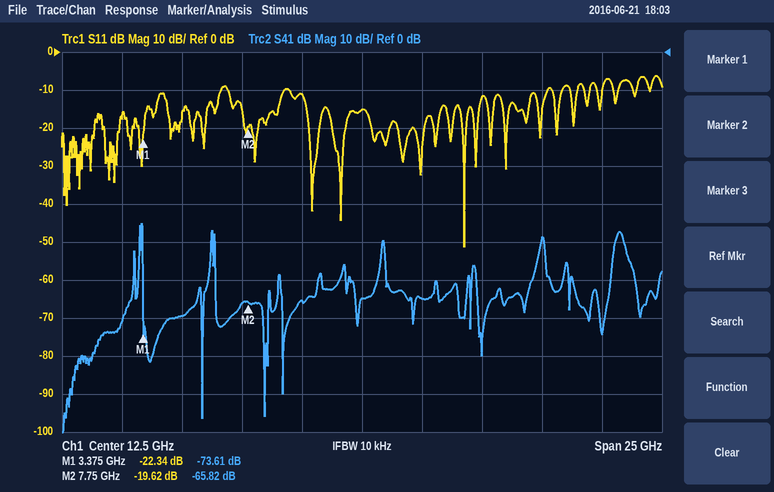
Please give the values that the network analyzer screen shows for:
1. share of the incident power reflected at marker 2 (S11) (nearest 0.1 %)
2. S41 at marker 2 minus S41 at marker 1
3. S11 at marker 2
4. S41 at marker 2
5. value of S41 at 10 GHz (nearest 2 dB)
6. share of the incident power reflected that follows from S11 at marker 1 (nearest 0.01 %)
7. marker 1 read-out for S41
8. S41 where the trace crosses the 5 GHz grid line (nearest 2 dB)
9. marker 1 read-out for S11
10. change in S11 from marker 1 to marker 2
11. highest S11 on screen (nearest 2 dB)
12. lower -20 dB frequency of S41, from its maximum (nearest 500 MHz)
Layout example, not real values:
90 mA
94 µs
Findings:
1.1 %
7.79 dB
-19.62 dB
-65.82 dB
-66 dB
0.58 %
-73.61 dB
-70 dB
-22.34 dB
2.72 dB
-6 dB
3.0 GHz
